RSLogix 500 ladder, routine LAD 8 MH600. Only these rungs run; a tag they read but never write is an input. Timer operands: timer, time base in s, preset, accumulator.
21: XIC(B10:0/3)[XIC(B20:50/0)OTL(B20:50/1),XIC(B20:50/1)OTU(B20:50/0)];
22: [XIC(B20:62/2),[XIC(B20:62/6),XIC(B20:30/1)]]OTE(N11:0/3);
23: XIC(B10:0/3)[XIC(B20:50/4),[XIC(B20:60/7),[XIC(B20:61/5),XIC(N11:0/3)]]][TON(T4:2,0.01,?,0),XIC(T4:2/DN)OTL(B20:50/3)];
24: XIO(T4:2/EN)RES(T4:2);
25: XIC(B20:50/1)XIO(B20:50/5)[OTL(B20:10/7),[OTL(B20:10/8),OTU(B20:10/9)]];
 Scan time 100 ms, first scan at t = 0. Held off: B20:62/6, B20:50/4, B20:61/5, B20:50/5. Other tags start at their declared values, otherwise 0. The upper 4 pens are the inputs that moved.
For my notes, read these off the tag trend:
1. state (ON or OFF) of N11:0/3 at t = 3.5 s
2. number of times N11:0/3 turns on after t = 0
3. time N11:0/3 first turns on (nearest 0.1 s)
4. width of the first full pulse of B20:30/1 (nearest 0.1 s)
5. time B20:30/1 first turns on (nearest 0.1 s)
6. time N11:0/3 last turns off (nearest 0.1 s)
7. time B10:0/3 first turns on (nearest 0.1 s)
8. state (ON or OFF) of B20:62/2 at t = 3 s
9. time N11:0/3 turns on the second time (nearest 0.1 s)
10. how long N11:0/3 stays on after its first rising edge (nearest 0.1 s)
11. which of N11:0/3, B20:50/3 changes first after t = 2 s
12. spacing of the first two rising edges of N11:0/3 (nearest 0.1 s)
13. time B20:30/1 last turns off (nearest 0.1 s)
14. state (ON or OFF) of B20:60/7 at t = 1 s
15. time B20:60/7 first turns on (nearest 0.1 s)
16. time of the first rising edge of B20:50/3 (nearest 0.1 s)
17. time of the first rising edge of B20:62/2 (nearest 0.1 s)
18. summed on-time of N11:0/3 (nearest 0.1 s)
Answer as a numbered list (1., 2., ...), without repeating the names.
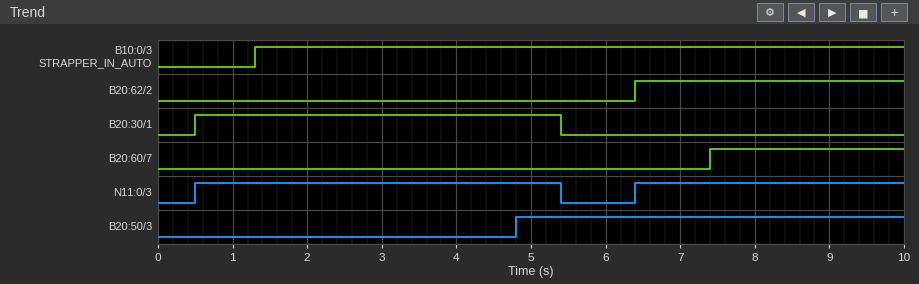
1. ON
2. 2
3. 0.5 s
4. 4.9 s
5. 0.5 s
6. 5.4 s
7. 1.3 s
8. OFF
9. 6.4 s
10. 4.9 s
11. B20:50/3
12. 5.9 s
13. 5.4 s
14. OFF
15. 7.4 s
16. 4.8 s
17. 6.4 s
18. 8.5 s
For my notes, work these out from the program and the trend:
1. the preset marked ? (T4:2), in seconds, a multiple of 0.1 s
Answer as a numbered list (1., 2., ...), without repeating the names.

1. 3.5 s
